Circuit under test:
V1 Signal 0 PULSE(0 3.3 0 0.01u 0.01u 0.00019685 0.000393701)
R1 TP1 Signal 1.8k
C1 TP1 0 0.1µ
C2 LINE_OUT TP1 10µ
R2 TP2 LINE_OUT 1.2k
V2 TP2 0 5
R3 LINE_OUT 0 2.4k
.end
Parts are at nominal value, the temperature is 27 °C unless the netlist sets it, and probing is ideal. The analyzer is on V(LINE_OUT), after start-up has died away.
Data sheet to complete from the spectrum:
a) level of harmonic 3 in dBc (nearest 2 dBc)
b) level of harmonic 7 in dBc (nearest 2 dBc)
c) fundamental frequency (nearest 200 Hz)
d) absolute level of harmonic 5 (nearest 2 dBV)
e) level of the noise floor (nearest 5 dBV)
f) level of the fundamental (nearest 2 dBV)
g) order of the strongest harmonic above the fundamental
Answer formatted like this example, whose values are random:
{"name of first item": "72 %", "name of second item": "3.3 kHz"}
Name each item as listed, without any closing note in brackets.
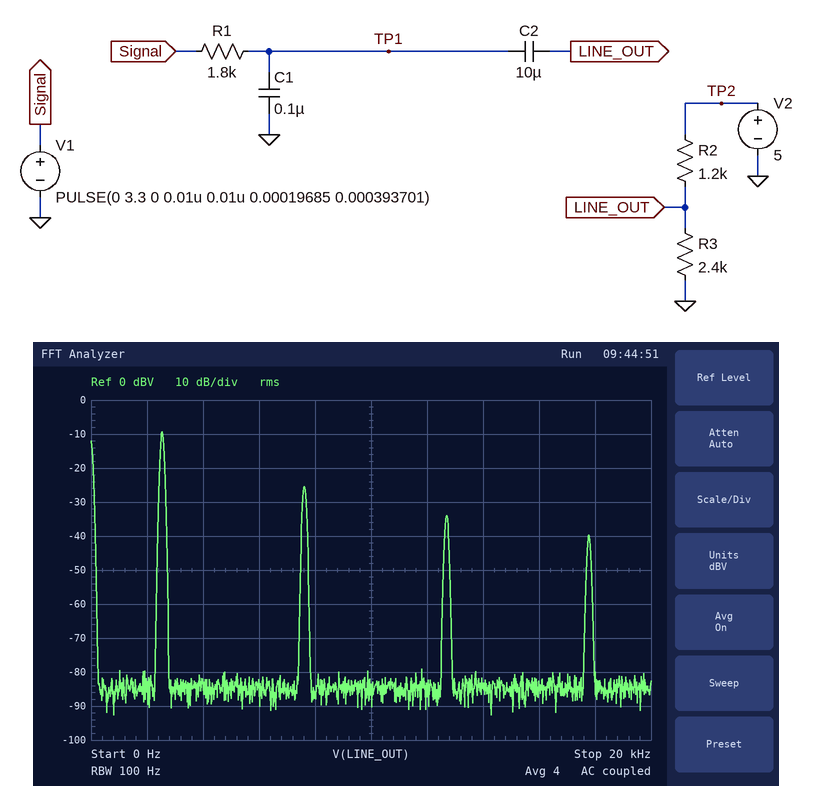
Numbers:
{"level of harmonic 3 in dBc": "-16 dBc", "level of harmonic 7 in dBc": "-30 dBc", "fundamental frequency": "2.6 kHz", "absolute level of harmonic 5": "-34 dBV", "level of the noise floor": "-85 dBV", "level of the fundamental": "-10 dBV", "order of the strongest harmonic above the fundamental": "3"}
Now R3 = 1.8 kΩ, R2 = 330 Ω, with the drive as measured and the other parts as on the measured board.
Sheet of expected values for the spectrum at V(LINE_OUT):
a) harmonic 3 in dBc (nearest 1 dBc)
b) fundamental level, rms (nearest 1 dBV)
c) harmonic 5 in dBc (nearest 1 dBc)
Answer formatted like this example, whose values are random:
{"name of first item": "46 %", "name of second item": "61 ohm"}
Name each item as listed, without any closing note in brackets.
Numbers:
{"harmonic 3 in dBc": "-13 dBc", "fundamental level, rms": "-15 dBV", "harmonic 5 in dBc": "-20 dBc"}
